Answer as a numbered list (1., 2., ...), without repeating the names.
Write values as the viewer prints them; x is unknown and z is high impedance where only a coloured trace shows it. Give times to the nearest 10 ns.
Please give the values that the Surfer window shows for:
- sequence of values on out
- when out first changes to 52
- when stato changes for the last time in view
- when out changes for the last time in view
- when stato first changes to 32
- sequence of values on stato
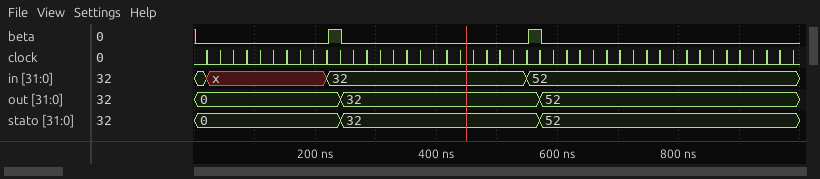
1. 0, 32, 52
2. 570 ns
3. 570 ns
4. 570 ns
5. 240 ns
6. 0, 32, 52
